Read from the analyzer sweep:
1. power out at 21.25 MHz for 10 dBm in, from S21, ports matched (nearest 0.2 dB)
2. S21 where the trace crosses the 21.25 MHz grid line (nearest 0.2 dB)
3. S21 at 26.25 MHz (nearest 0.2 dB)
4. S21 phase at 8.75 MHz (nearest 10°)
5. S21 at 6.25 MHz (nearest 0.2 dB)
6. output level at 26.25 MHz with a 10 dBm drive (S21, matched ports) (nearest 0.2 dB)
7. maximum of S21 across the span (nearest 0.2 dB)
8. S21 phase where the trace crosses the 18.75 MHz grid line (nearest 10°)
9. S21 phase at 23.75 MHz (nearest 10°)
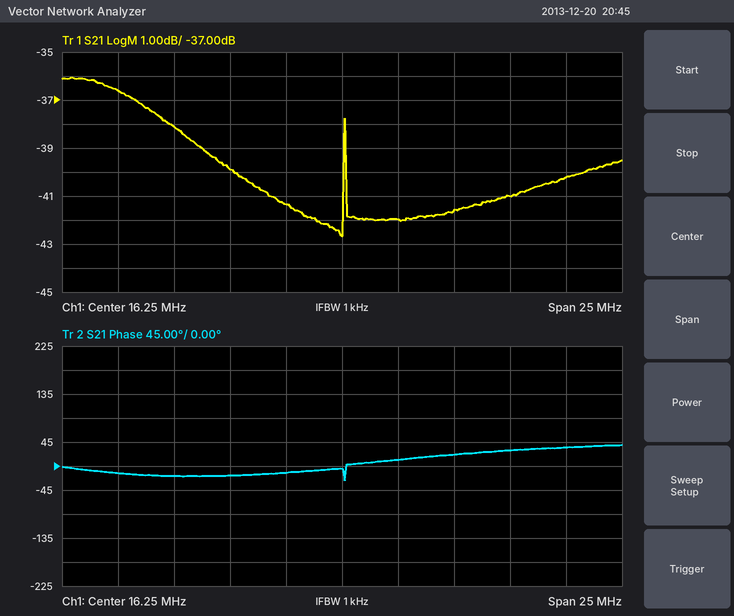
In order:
-31.6 dBm
-41.6 dB
-40.2 dB
-20°
-36.6 dB
-30.2 dBm
-36.0 dB
10°
30°
